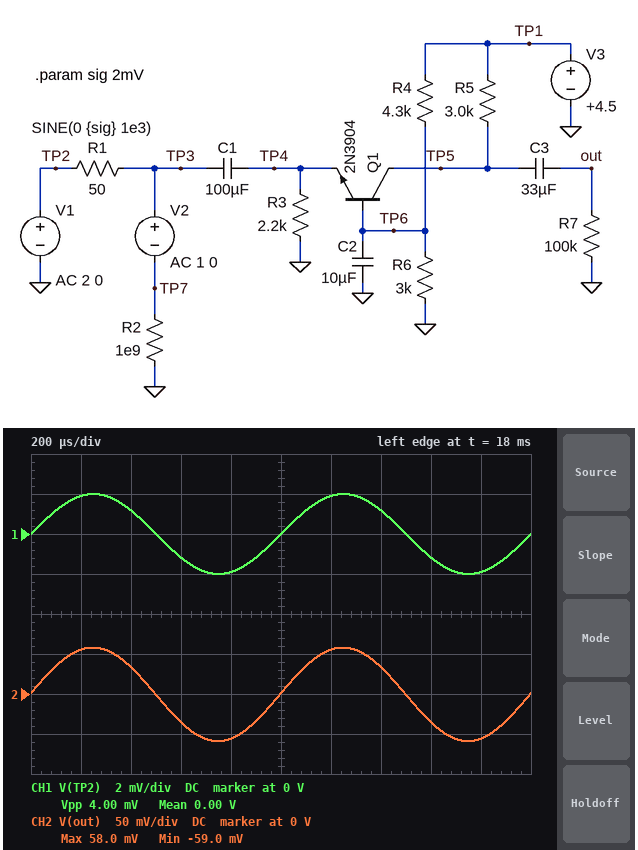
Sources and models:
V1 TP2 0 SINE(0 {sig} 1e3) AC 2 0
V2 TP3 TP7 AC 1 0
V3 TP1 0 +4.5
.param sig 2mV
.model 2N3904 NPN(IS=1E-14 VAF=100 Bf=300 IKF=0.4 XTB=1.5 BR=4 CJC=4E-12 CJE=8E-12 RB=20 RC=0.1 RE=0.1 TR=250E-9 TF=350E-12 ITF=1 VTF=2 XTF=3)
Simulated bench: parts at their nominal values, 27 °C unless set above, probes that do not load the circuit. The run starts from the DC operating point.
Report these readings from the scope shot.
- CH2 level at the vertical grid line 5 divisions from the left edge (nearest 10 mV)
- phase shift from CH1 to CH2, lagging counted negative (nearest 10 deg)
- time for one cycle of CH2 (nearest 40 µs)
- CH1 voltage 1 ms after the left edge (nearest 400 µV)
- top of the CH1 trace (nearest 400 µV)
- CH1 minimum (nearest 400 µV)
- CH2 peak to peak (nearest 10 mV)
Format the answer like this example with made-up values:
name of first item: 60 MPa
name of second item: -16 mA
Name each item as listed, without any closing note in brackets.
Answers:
CH2 level at the vertical grid line 5 divisions from the left edge: 0 V
phase shift from CH1 to CH2, lagging counted negative: 0 deg
time for one cycle of CH2: 1.00 ms
CH1 voltage 1 ms after the left edge: 0 V
top of the CH1 trace: 2.0 mV
CH1 minimum: -2.0 mV
CH2 peak to peak: 120 mV
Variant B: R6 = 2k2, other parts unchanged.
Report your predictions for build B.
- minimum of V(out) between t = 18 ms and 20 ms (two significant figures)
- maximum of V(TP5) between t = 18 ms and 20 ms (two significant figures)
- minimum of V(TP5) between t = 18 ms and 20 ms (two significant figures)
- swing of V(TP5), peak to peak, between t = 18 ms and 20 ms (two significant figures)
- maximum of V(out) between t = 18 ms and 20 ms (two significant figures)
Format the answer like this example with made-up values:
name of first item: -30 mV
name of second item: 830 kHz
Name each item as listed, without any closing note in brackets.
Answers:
minimum of V(out) between t = 18 ms and 20 ms: -50 mV
maximum of V(TP5) between t = 18 ms and 20 ms: 3.3 V
minimum of V(TP5) between t = 18 ms and 20 ms: 3.2 V
swing of V(TP5), peak to peak, between t = 18 ms and 20 ms: 100 mV
maximum of V(out) between t = 18 ms and 20 ms: 49 mV
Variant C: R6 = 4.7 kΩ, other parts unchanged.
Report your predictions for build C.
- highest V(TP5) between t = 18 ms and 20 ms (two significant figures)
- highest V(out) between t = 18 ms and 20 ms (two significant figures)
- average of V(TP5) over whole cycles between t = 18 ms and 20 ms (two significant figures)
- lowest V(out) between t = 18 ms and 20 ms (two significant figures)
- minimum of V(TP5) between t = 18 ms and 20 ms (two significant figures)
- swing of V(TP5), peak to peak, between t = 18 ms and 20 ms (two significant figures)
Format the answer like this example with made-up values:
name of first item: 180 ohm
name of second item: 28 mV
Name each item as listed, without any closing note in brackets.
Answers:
highest V(TP5) between t = 18 ms and 20 ms: 2.3 V
highest V(out) between t = 18 ms and 20 ms: 68 mV
average of V(TP5) over whole cycles between t = 18 ms and 20 ms: 2.2 V
lowest V(out) between t = 18 ms and 20 ms: -68 mV
minimum of V(TP5) between t = 18 ms and 20 ms: 2.1 V
swing of V(TP5), peak to peak, between t = 18 ms and 20 ms: 140 mV
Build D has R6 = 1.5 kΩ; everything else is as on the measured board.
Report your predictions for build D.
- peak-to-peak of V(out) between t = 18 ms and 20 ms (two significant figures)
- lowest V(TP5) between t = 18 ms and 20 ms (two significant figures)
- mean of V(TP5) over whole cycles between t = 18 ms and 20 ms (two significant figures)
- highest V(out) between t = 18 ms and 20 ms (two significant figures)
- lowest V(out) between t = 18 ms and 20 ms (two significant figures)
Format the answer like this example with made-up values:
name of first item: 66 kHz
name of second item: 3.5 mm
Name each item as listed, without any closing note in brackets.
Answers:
peak-to-peak of V(out) between t = 18 ms and 20 ms: 74 mV
lowest V(TP5) between t = 18 ms and 20 ms: 3.7 V
mean of V(TP5) over whole cycles between t = 18 ms and 20 ms: 3.8 V
highest V(out) between t = 18 ms and 20 ms: 36 mV
lowest V(out) between t = 18 ms and 20 ms: -37 mV
